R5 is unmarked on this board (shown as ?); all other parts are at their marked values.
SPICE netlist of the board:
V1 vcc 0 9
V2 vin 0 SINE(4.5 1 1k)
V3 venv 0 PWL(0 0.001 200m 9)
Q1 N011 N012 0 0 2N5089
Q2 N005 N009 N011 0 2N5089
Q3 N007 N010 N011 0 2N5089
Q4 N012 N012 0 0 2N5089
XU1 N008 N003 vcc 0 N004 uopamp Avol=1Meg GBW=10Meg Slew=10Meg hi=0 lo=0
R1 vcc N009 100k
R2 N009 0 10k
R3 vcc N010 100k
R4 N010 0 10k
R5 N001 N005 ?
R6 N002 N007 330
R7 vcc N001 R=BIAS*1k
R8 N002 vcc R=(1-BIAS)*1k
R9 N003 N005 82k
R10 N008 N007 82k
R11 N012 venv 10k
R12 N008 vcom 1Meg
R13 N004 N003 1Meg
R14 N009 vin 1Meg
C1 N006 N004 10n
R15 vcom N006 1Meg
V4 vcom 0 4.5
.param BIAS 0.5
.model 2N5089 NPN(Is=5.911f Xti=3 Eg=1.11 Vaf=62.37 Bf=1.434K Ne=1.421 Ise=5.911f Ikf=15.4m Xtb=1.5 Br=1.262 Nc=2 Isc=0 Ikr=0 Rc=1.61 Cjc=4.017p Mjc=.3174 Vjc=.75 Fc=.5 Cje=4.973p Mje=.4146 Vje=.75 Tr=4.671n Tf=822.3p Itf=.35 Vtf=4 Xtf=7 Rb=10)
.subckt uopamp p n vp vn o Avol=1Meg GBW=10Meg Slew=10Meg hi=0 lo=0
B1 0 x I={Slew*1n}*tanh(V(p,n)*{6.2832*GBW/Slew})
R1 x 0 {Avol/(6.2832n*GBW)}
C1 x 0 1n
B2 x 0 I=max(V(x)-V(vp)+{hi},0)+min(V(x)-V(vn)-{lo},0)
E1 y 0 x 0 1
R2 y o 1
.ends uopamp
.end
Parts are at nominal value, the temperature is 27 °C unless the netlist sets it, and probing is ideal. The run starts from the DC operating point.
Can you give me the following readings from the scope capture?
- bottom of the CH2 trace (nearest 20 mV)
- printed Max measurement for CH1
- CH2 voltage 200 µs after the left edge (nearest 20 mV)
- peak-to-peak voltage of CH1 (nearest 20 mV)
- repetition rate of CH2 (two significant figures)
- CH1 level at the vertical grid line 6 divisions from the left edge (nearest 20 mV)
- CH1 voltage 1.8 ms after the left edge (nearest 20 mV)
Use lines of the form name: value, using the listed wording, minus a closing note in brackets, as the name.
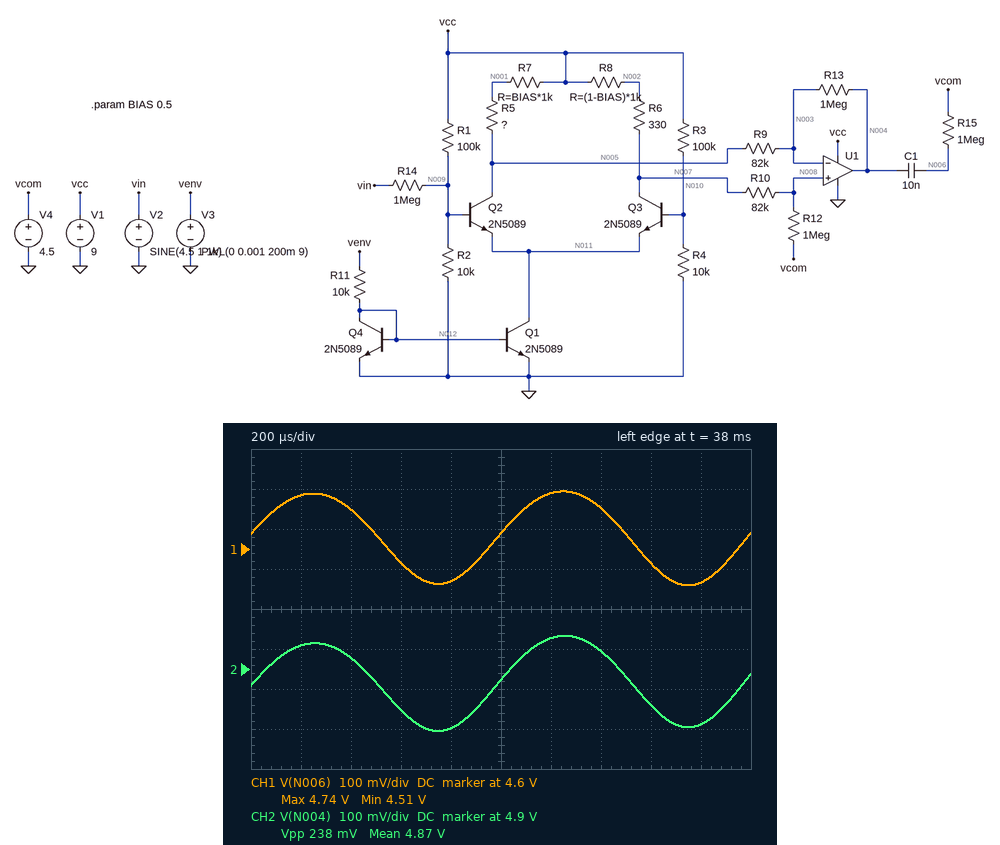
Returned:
bottom of the CH2 trace: 4.74 V
printed Max measurement for CH1: 4.74 V
CH2 voltage 200 µs after the left edge: 4.96 V
peak-to-peak voltage of CH1: 240 mV
repetition rate of CH2: 1.0 kHz
CH1 level at the vertical grid line 6 divisions from the left edge: 4.74 V
CH1 voltage 1.8 ms after the left edge: 4.52 V
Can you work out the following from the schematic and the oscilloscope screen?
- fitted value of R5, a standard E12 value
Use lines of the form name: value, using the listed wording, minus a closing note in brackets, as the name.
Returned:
fitted value of R5, a standard E12 value: 100 Ω
